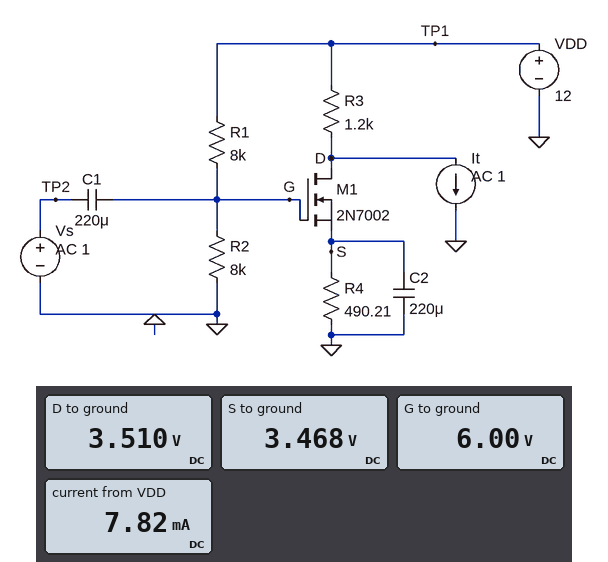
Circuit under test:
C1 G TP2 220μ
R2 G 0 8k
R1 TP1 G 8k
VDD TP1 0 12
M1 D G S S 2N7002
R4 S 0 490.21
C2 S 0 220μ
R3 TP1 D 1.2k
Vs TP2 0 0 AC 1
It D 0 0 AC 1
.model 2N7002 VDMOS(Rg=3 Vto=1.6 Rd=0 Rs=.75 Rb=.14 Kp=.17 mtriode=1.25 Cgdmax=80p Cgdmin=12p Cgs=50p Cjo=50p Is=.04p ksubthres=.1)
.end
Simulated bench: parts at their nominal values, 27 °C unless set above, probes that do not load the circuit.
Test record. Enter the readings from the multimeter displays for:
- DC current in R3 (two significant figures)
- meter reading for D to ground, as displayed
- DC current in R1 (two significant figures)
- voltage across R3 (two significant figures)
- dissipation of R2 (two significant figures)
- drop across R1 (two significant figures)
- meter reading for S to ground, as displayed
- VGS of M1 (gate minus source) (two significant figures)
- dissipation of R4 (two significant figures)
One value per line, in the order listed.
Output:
7.1 mA
3.510 V
750 µA
8.5 V
4.5 mW
6.0 V
3.468 V
2.5 V
25 mW
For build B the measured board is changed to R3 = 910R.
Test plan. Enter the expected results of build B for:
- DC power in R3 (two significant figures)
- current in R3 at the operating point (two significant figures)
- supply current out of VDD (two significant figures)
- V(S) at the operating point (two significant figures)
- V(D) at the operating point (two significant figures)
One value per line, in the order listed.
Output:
63 mW
8.3 mA
9.1 mA
4.1 V
4.4 V
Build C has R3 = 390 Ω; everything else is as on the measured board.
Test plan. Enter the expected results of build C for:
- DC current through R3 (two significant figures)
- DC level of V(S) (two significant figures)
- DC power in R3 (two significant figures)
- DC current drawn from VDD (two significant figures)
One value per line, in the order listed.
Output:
8.3 mA
4.1 V
27 mW
9.1 mA
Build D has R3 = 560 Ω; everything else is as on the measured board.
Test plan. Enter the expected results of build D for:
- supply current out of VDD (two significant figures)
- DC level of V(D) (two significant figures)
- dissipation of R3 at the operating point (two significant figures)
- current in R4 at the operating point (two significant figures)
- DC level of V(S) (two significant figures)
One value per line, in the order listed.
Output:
9.1 mA
7.3 V
39 mW
8.3 mA
4.1 V
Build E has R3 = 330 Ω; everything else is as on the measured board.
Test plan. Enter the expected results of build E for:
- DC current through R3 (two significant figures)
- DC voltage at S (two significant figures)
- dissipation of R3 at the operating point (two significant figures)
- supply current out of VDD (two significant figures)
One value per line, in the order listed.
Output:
8.3 mA
4.1 V
23 mW
9.1 mA
